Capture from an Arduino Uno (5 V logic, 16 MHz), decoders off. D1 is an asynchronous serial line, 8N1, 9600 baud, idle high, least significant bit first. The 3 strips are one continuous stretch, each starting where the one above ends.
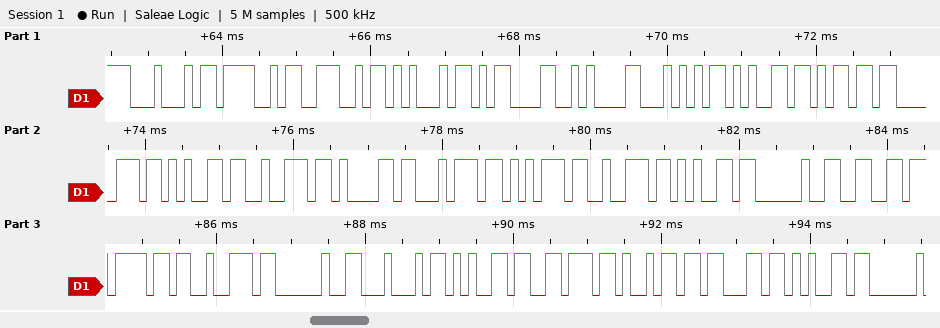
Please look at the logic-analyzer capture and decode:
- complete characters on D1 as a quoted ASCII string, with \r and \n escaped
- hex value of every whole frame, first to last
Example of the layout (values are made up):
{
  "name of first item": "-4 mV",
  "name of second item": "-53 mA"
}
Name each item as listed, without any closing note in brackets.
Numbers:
{
  "complete characters on D1 as a quoted ASCII string, with \\r and \\n escaped": "\"DONE\\r\\nTemperature for Device\"",
  "hex value of every whole frame, first to last": "0x44 0x4F 0x4E 0x45 0x0D 0x0A 0x54 0x65 0x6D 0x70 0x65 0x72 0x61 0x74 0x75 0x72 0x65 0x20 0x66 0x6F 0x72 0x20 0x44 0x65 0x76 0x69 0x63 0x65"
}
